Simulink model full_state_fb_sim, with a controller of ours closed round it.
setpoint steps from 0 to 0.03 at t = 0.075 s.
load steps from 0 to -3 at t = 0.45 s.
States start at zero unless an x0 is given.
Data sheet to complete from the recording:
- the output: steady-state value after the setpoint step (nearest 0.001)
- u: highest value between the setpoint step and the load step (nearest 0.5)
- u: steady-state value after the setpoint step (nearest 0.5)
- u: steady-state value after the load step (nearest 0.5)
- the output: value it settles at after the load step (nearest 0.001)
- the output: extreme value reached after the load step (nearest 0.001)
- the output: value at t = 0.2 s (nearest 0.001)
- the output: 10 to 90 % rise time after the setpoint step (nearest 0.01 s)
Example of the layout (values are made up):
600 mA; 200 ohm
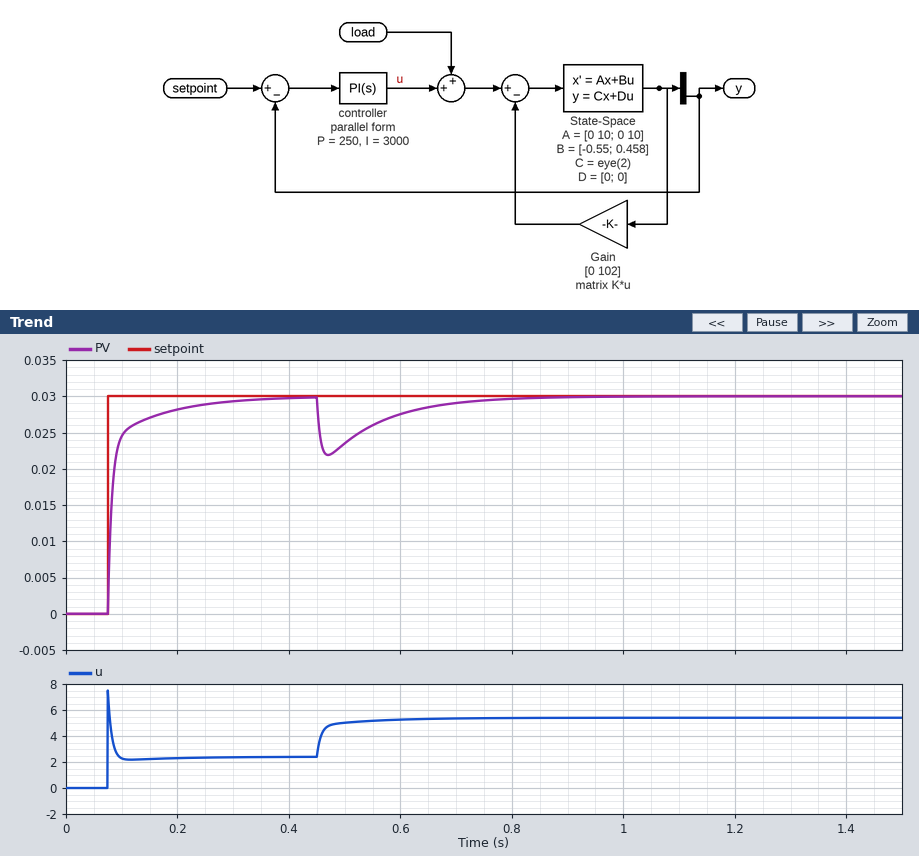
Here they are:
0.030; 7.5; 2.5; 5.5; 0.030; 0.022; 0.028; 0.07 s
